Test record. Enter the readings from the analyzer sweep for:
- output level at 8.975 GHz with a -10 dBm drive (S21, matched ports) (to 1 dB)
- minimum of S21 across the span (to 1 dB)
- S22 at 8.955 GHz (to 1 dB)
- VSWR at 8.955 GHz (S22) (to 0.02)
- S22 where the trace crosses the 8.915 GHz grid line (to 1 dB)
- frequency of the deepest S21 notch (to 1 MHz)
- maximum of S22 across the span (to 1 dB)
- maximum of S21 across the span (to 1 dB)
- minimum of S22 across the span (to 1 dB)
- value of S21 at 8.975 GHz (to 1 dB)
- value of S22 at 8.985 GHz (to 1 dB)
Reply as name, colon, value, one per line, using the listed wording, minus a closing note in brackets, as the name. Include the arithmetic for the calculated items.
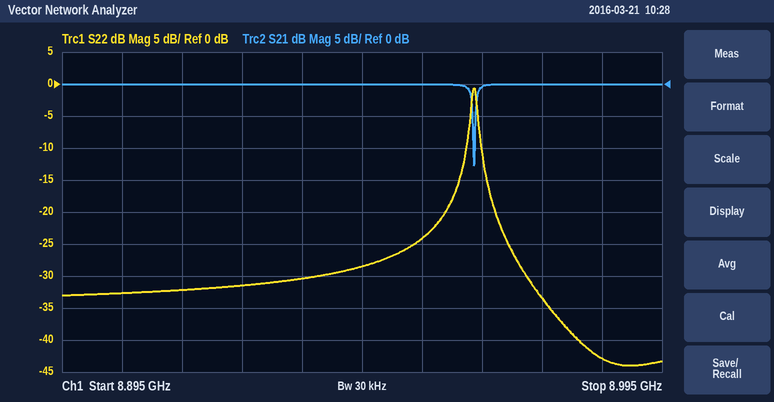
output level at 8.975 GHz with a -10 dBm drive (S21, matched ports): -10 dBm + (0 dB) = -10 dBm
minimum of S21 across the span: -13 dB
S22 at 8.955 GHz: -24 dB
VSWR at 8.955 GHz (S22): |Γ| = 10^(-24/20) = 0.0631; VSWR = (1 + 0.0631)/(1 − 0.0631) ≈ 1.13, so 1.14 to the nearest 0.02
S22 where the trace crosses the 8.915 GHz grid line: -32 dB
frequency of the deepest S21 notch: 8.964 GHz
maximum of S22 across the span: -1 dB
maximum of S21 across the span: 0 dB
minimum of S22 across the span: -44 dB
value of S21 at 8.975 GHz: 0 dB
value of S22 at 8.985 GHz: -43 dB
